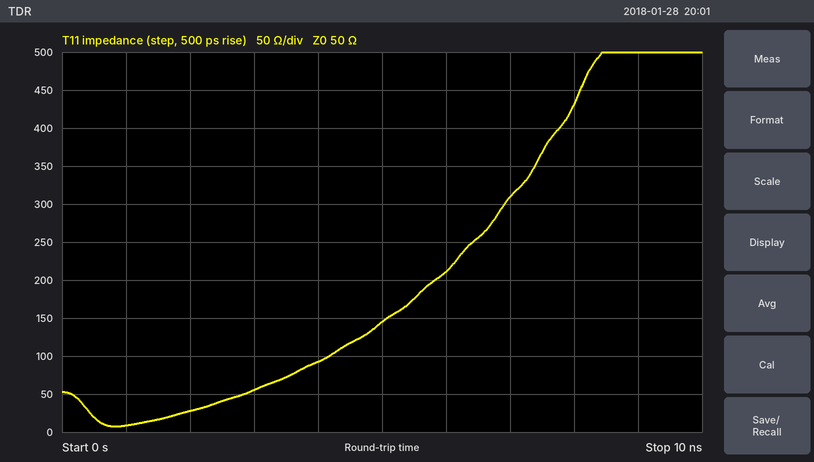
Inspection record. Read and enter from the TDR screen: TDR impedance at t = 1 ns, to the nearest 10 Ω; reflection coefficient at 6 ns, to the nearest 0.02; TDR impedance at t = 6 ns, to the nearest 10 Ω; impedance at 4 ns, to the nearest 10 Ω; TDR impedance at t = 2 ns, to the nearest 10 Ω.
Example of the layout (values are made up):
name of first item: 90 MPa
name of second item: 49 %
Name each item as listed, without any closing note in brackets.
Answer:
TDR impedance at t = 1 ns, to the nearest 10 Ω: 10 Ω
reflection coefficient at 6 ns, to the nearest 0.02: +0.62
TDR impedance at t = 6 ns, to the nearest 10 Ω: 210 Ω
impedance at 4 ns, to the nearest 10 Ω: 90 Ω
TDR impedance at t = 2 ns, to the nearest 10 Ω: 30 Ω
